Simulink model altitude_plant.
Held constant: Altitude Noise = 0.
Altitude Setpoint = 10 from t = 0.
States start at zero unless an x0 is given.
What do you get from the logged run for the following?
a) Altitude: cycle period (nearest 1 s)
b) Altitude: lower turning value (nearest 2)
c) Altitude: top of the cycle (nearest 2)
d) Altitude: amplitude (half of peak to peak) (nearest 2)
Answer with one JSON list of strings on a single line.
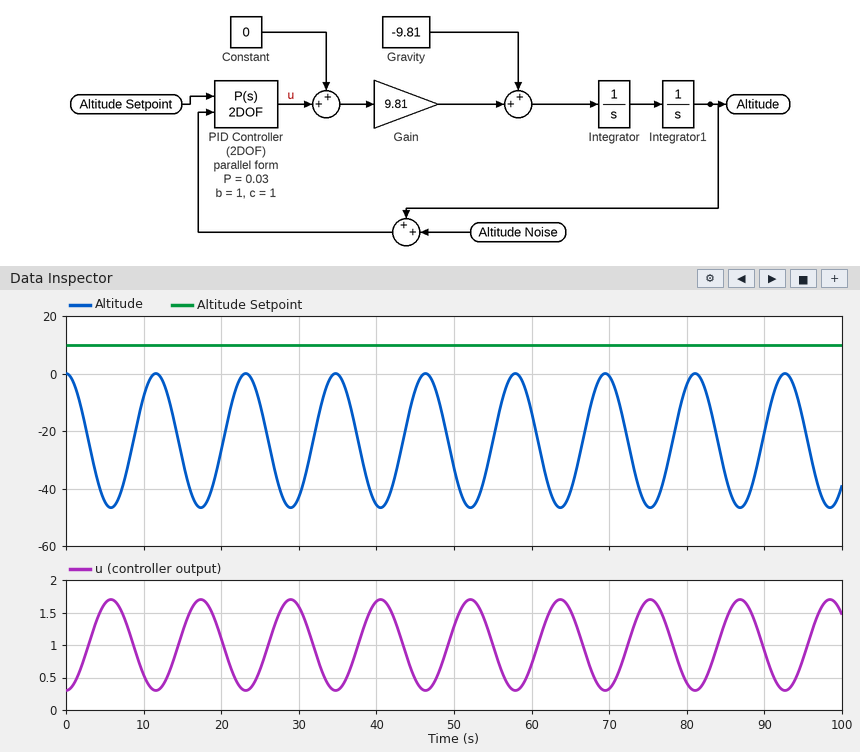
["12 s", "-46", "0", "24"]
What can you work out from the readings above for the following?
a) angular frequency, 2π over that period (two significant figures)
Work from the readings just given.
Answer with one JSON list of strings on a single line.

["0.52 rad/s"]
